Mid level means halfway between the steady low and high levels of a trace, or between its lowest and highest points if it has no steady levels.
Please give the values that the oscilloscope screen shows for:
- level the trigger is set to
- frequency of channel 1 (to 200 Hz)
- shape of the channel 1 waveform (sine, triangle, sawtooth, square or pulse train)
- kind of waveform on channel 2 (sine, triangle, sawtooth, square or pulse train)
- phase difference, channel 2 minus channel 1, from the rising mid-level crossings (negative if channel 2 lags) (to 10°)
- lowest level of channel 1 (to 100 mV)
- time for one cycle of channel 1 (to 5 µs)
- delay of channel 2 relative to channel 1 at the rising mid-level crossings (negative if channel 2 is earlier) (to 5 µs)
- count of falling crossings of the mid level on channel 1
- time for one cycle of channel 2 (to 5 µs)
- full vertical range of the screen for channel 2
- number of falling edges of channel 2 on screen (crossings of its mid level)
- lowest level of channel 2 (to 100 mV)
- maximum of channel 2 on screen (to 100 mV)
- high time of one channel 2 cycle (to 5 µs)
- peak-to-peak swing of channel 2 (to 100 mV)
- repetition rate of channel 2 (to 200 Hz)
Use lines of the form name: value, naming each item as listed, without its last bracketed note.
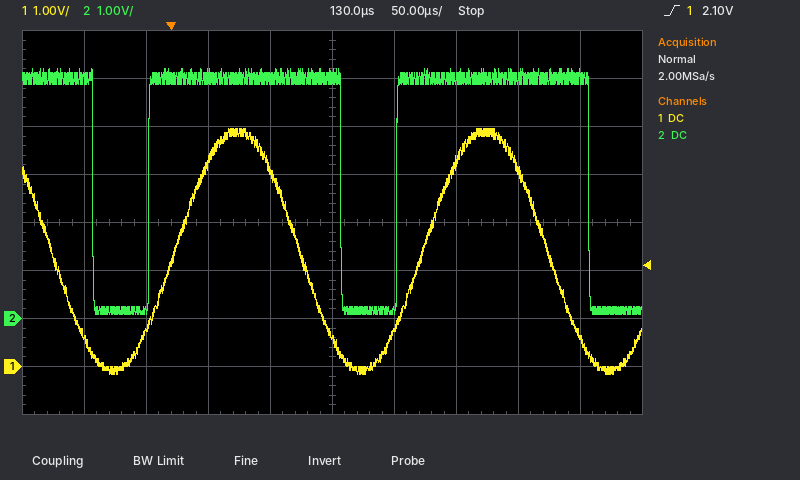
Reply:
level the trigger is set to: 2.10 V
frequency of channel 1: 5.0 kHz
shape of the channel 1 waveform: sine
kind of waveform on channel 2: pulse train
phase difference, channel 2 minus channel 1, from the rising mid-level crossings (negative if channel 2 lags): +40°
lowest level of channel 1: -200 mV
time for one cycle of channel 1: 200 µs
delay of channel 2 relative to channel 1 at the rising mid-level crossings (negative if channel 2 is earlier): -20 µs
count of falling crossings of the mid level on channel 1: 3
time for one cycle of channel 2: 200 µs
full vertical range of the screen for channel 2: 8 V
number of falling edges of channel 2 on screen: 3
lowest level of channel 2: 100 mV
maximum of channel 2 on screen: 5.2 V
high time of one channel 2 cycle: 155 µs
peak-to-peak swing of channel 2: 5.1 V
repetition rate of channel 2: 5.0 kHz
